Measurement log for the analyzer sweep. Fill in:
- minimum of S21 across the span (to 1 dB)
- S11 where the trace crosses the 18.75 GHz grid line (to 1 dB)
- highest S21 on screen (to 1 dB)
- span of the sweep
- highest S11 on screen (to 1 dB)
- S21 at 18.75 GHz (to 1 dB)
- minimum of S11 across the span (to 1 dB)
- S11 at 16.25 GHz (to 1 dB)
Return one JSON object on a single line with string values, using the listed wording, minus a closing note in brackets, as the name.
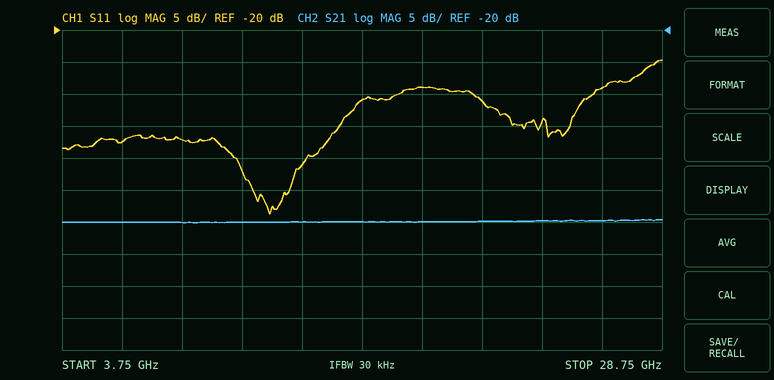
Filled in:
{"minimum of S21 across the span": "-50 dB", "S11 where the trace crosses the 18.75 GHz grid line": "-29 dB", "highest S21 on screen": "-50 dB", "span of the sweep": "25 GHz", "highest S11 on screen": "-25 dB", "S21 at 18.75 GHz": "-50 dB", "minimum of S11 across the span": "-49 dB", "S11 at 16.25 GHz": "-31 dB"}
